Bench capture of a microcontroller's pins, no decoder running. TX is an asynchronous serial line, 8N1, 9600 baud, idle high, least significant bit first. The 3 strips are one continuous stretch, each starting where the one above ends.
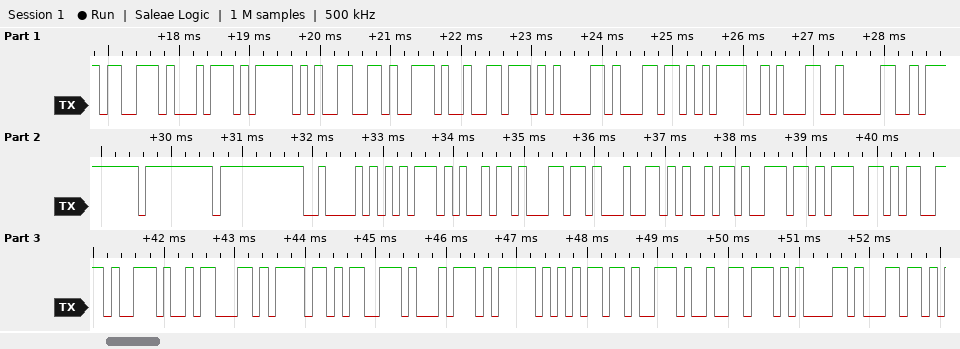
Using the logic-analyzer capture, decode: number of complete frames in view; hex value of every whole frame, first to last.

34
73 74 5F 66 2E 76 61 6C 3D 31 30 FF FF FF 42 75 69 6C 64 69 6E 67 73 2E 63 6F 73 74 5F 6D 2E 76 61 6C
